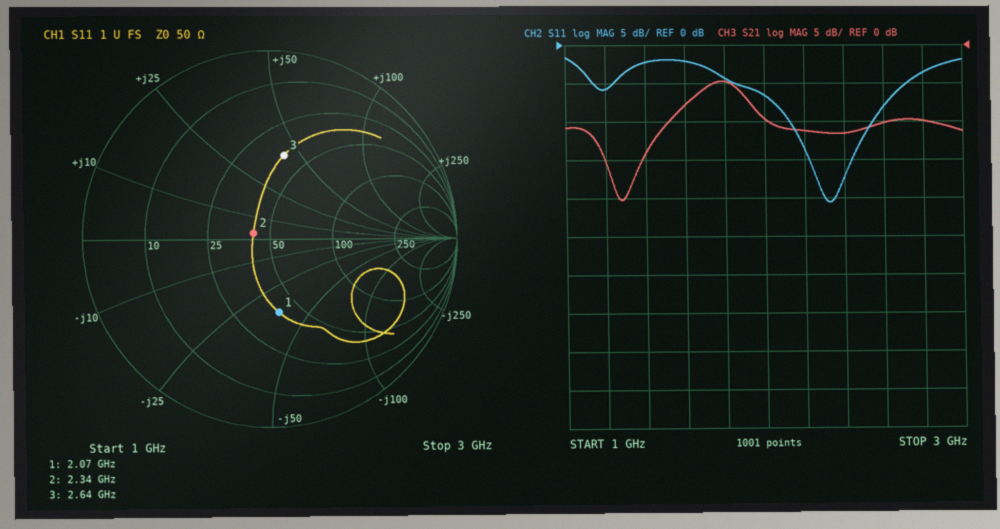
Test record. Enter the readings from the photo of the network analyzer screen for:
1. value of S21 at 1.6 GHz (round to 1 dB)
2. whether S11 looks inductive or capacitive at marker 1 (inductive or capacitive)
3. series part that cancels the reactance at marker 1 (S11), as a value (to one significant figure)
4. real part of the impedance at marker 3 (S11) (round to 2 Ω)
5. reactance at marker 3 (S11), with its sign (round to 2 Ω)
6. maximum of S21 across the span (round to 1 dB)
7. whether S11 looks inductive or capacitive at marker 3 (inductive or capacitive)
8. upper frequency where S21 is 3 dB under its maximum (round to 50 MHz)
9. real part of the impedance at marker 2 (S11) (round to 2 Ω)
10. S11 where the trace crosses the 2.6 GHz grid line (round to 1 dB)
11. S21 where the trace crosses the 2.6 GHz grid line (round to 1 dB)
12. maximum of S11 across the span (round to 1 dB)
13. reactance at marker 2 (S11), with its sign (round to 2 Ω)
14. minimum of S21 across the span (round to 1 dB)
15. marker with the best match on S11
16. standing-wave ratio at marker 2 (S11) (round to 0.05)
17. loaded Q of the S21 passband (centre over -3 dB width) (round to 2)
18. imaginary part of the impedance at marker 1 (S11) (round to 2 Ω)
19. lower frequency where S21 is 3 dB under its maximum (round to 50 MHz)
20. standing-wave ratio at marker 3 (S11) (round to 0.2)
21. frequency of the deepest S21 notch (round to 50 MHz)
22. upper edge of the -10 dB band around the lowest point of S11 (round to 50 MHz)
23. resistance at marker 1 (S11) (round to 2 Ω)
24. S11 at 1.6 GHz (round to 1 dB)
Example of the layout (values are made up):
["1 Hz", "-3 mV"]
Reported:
["-8 dB", "capacitive", "3 nH", "38 Ω", "+42 Ω", "-5 dB", "inductive", "1.95 GHz", "42 Ω", "-8 dB", "-10 dB", "-2 dB", "+2 Ω", "-20 dB", "marker 2", "1.20", "6", "-36 Ω", "1.60 GHz", "2.6", "1.30 GHz", "2.55 GHz", "40 Ω", "-2 dB"]
